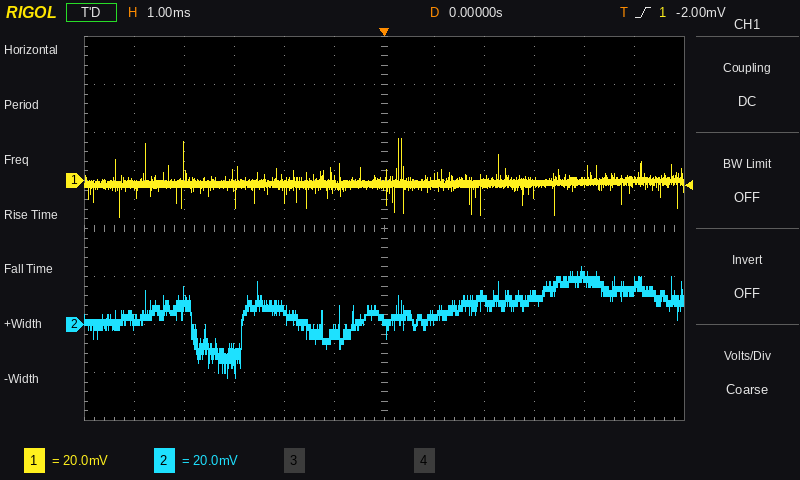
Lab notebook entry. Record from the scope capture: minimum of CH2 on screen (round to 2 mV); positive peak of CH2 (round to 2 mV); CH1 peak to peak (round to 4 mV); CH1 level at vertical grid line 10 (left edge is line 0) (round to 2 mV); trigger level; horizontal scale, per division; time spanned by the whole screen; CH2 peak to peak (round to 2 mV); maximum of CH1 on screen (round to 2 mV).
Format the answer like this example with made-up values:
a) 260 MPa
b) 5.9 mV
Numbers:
a) -22 mV
b) 24 mV
c) 32 mV
d) 0 mV
e) -2.00 mV
f) 1 ms
g) 12 ms
h) 46 mV
i) 18 mV
